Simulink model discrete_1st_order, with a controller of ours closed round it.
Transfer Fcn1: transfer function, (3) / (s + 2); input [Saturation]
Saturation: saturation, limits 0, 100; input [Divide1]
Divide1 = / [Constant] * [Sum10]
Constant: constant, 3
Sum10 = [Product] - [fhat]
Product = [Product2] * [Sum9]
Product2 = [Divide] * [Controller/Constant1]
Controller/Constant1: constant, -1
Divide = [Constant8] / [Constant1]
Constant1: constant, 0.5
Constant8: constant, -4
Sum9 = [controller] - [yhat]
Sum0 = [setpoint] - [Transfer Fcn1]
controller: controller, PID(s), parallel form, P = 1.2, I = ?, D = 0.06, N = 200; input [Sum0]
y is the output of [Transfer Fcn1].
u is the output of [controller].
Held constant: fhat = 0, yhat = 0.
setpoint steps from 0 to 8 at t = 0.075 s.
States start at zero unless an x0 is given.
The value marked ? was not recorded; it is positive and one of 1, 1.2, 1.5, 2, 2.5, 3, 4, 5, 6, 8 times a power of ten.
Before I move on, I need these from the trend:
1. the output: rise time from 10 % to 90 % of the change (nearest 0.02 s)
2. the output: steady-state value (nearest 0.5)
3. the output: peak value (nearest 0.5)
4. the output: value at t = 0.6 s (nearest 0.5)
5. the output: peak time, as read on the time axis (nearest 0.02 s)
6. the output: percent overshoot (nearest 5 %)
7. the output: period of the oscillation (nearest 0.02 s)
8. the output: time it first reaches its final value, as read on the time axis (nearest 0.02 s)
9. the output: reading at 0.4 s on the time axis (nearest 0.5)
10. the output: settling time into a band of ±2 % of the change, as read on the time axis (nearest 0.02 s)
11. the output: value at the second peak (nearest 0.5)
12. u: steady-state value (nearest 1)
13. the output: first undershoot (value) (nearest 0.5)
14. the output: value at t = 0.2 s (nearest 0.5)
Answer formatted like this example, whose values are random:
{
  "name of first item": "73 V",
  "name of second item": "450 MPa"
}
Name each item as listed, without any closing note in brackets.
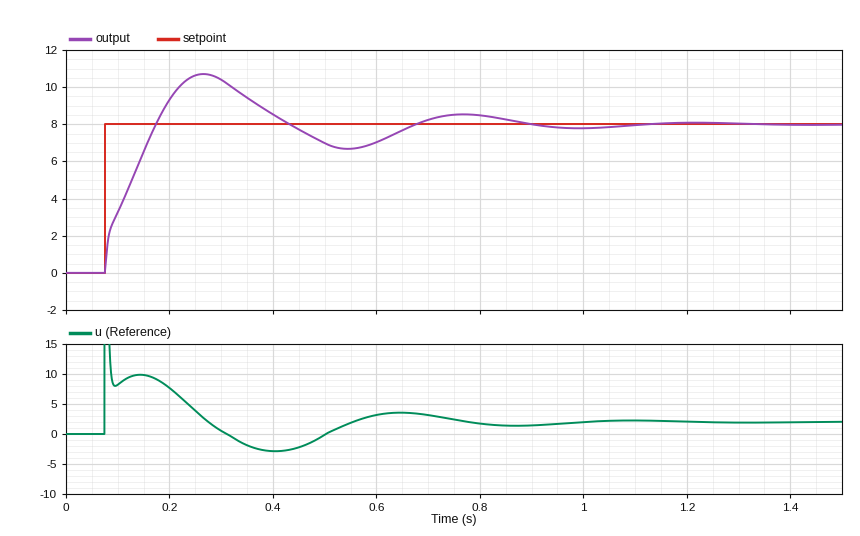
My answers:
{
  "the output: rise time from 10 % to 90 % of the change": "0.08 s",
  "the output: steady-state value": "8.0",
  "the output: peak value": "10.5",
  "the output: value at t = 0.6 s": "7.0",
  "the output: peak time, as read on the time axis": "0.26 s",
  "the output: percent overshoot": "35 %",
  "the output: period of the oscillation": "0.50 s",
  "the output: time it first reaches its final value, as read on the time axis": "0.18 s",
  "the output: reading at 0.4 s on the time axis": "8.5",
  "the output: settling time into a band of ±2 % of the change, as read on the time axis": "1.04 s",
  "the output: value at the second peak": "8.5",
  "u: steady-state value": "2",
  "the output: first undershoot (value)": "6.5",
  "the output: value at t = 0.2 s": "9.5"
}
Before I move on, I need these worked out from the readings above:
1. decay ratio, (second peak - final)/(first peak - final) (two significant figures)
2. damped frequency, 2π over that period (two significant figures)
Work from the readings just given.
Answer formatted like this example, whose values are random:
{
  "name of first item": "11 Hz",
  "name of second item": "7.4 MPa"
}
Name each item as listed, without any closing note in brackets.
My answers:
{
  "decay ratio, (second peak - final)/(first peak - final)": "0.20",
  "damped frequency, 2π over that period": "13 rad/s"
}
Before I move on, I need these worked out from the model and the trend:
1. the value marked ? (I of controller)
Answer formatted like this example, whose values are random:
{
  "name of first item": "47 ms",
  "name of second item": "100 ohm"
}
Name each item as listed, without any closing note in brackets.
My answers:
{
  "the value marked ?": "40"
}
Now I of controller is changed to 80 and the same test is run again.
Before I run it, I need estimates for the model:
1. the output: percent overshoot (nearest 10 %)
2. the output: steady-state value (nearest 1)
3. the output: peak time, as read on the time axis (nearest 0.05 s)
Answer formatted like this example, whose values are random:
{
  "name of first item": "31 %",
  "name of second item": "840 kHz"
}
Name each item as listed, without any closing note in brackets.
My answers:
{
  "the output: percent overshoot": "40 %",
  "the output: steady-state value": "8",
  "the output: peak time, as read on the time axis": "0.20 s"
}
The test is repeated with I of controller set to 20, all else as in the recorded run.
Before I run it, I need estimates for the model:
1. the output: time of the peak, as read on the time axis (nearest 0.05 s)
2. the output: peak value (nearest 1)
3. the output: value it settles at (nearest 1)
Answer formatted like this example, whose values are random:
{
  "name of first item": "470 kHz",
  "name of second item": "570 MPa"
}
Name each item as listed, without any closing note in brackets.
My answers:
{
  "the output: time of the peak, as read on the time axis": "0.35 s",
  "the output: peak value": "10",
  "the output: value it settles at": "8"
}
